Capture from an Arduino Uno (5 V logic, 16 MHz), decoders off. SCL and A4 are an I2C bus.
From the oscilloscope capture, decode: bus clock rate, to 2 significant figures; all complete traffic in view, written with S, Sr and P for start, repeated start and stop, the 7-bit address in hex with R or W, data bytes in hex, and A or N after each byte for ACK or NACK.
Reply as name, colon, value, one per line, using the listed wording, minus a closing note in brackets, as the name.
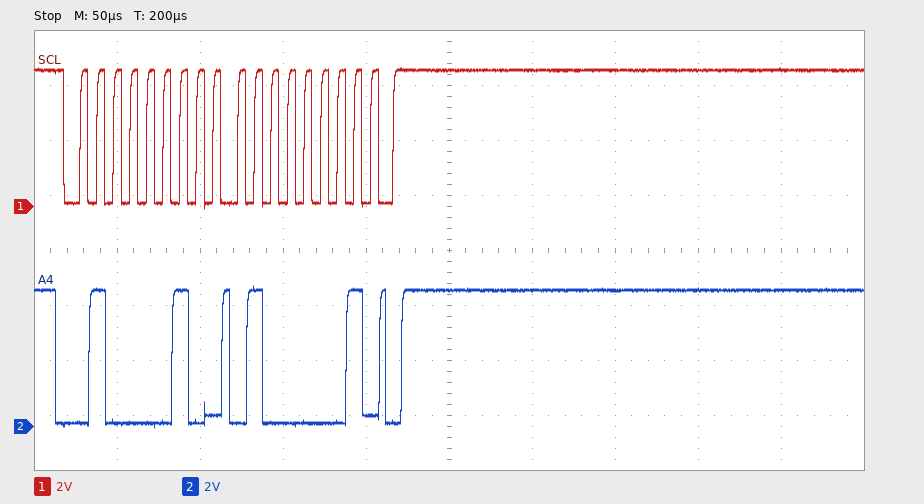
bus clock rate, to 2 significant figures: 100 kHz
all complete traffic in view, written with S, Sr and P for start, repeated start and stop, the 7-bit address in hex with R or W, data bytes in hex, and A or N after each byte for ACK or NACK: S 21W A 41 A P
